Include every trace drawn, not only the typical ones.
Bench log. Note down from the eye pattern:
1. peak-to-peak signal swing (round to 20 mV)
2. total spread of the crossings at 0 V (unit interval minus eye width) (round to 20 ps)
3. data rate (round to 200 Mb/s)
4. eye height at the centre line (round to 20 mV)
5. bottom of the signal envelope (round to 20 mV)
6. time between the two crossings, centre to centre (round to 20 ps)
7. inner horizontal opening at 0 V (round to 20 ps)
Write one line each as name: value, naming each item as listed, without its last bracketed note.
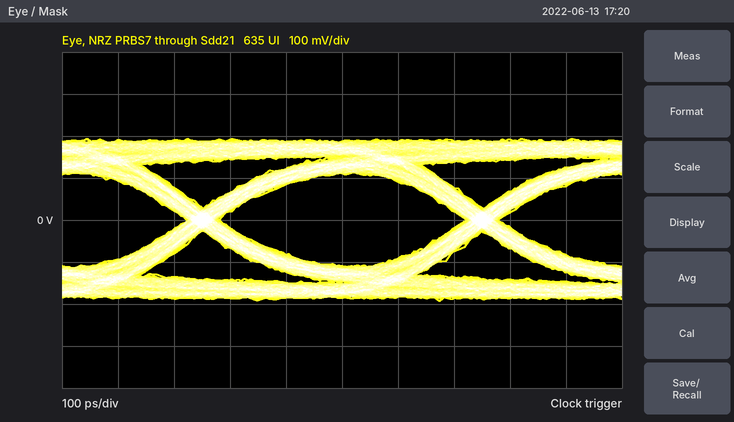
peak-to-peak signal swing: 380 mV
total spread of the crossings at 0 V (unit interval minus eye width): 60 ps
data rate: 2.0 Gb/s
eye height at the centre line: 220 mV
bottom of the signal envelope: -200 mV
time between the two crossings, centre to centre: 500 ps
inner horizontal opening at 0 V: 440 ps
